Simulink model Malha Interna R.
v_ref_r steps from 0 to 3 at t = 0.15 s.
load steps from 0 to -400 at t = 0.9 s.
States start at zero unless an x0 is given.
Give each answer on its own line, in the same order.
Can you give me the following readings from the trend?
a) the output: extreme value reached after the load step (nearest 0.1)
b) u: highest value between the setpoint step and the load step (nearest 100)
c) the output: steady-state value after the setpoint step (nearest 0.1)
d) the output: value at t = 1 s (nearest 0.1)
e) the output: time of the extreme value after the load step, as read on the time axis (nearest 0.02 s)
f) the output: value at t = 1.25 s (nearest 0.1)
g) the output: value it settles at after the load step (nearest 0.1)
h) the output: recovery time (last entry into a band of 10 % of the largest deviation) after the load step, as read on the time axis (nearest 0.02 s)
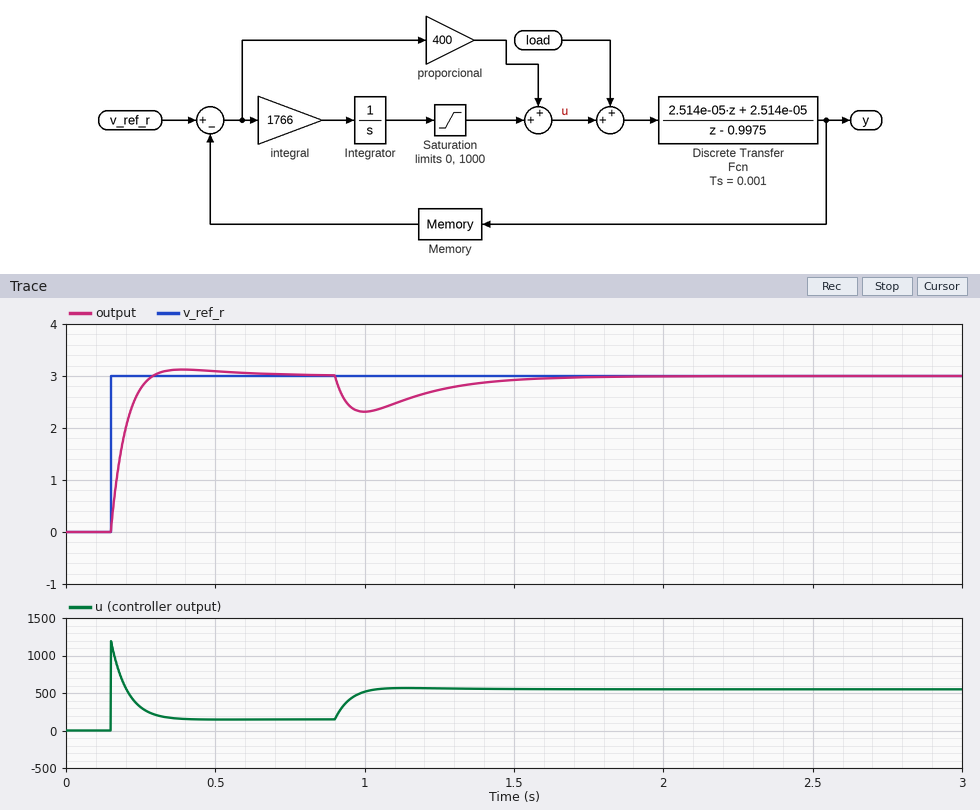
2.3
1200
3.0
2.3
1.00 s
2.7
3.0
1.52 s
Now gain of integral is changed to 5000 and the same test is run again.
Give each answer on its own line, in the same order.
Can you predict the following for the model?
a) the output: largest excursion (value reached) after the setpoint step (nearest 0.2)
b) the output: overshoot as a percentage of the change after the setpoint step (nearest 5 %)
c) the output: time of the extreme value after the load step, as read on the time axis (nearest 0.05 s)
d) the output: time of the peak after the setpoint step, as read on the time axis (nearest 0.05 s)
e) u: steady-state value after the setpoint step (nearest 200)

3.4
15 %
0.95 s
0.30 s
200
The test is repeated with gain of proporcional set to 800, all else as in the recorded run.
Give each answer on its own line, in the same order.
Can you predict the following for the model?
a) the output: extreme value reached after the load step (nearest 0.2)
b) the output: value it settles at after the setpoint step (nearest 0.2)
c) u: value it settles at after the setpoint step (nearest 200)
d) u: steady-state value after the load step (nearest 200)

2.6
3.0
200
600
